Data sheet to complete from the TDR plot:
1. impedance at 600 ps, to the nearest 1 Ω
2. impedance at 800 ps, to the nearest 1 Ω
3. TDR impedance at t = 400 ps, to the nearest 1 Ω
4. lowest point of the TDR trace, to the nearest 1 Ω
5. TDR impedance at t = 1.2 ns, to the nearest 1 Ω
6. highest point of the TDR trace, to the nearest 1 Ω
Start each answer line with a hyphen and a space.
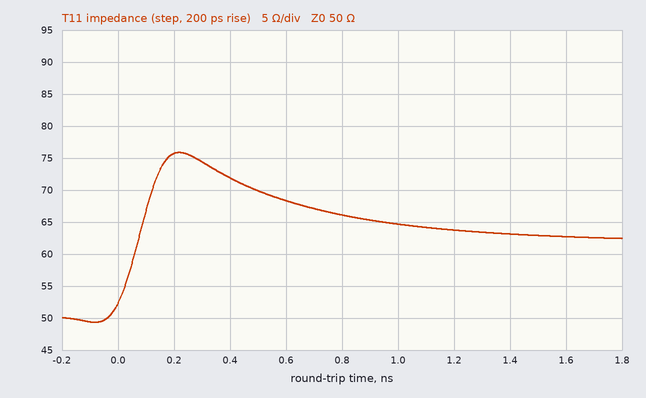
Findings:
- 68 Ω
- 66 Ω
- 72 Ω
- 49 Ω
- 64 Ω
- 76 Ω
